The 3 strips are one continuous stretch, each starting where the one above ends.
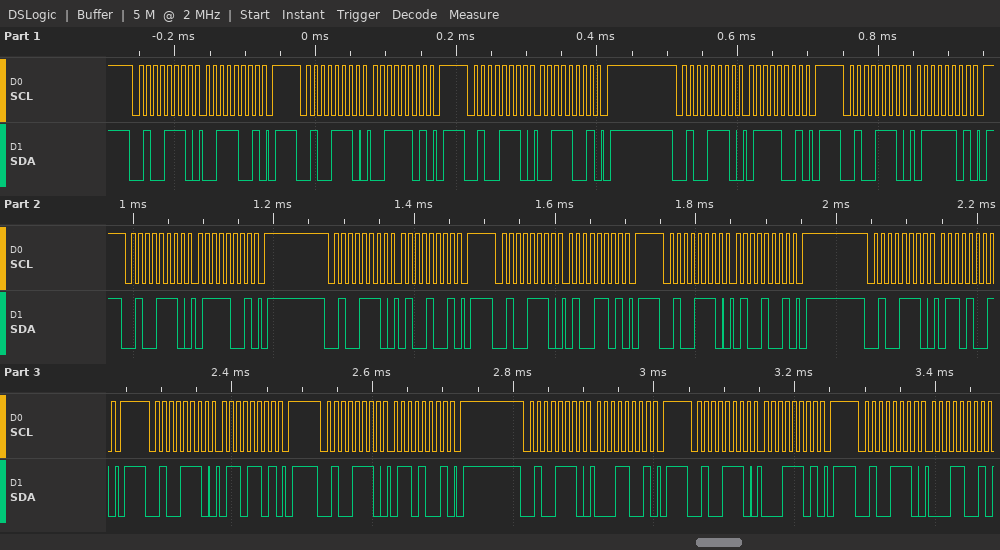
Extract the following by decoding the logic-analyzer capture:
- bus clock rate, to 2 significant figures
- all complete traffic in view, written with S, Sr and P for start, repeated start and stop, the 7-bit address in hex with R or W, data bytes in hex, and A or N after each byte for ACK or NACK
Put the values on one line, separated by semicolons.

100 kHz; S 27W A 39 A P S 27W A 3D A P S 27W A 39 A P S 27W A 79 A P S 27W A 7D A P S 27W A 79 A P S 27W A 49 A P S 27W A 4D A P S 27W A 49 A P S 27W A 69 A P S 27W A 6D A P S 27W A 69 A P S 27W A 19 A P S 27W A 1D A P S 27W A 19 A
